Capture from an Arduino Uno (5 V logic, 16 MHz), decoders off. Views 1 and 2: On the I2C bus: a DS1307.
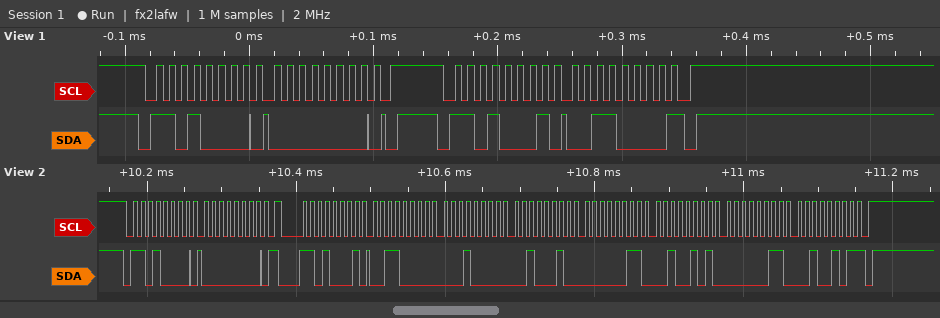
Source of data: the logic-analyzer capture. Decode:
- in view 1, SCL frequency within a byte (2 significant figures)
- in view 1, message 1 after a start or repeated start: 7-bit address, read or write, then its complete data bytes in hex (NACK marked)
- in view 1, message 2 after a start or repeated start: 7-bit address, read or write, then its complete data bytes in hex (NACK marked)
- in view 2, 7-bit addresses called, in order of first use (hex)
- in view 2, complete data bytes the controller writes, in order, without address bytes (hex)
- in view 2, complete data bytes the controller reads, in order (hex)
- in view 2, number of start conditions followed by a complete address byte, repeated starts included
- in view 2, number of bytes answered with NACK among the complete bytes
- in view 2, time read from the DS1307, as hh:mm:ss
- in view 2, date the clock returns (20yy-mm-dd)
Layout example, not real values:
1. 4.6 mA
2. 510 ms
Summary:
1. 100 kHz
2. 0x68 write: 00
3. 0x68 read: 30 NACK
4. 0x68
5. 00
6. 30 10 22 03 25 03 25
7. 2
8. 1
9. 22:10:30
10. 2025-03-25
